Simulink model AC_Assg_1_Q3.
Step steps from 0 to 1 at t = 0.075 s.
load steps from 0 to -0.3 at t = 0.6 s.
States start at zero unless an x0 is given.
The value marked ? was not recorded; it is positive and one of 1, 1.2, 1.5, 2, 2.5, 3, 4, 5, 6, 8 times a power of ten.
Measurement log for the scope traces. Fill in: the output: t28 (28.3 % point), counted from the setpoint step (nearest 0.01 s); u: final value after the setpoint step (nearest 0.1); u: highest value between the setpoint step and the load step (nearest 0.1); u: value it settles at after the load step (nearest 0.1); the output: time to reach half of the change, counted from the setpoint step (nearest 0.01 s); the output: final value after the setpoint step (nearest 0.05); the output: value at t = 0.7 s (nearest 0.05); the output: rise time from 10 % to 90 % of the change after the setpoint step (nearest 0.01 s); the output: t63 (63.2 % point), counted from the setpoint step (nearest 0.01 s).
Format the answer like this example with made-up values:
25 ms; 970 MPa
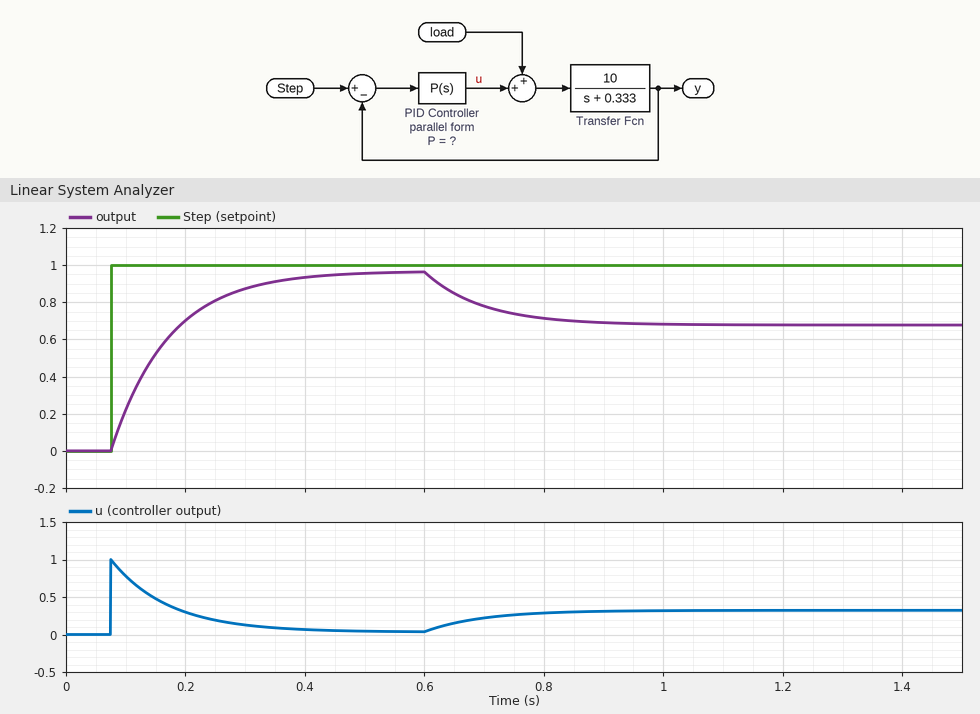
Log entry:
0.03 s; 0.0; 1.0; 0.3; 0.07 s; 0.95; 0.80; 0.21 s; 0.10 s
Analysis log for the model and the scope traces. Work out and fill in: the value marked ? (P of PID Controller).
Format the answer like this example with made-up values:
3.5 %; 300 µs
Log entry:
1
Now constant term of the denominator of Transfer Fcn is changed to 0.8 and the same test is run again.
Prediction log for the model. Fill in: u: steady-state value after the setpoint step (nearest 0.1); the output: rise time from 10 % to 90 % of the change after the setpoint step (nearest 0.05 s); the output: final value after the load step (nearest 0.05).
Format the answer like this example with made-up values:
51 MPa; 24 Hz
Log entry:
0.1; 0.20 s; 0.65
